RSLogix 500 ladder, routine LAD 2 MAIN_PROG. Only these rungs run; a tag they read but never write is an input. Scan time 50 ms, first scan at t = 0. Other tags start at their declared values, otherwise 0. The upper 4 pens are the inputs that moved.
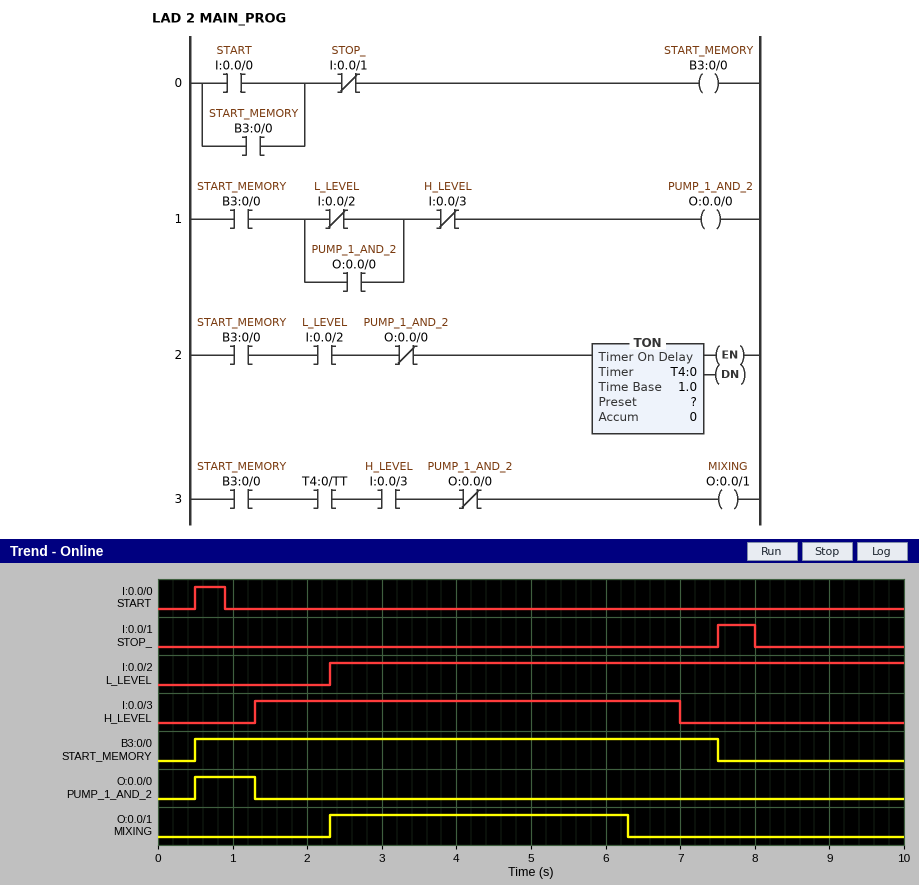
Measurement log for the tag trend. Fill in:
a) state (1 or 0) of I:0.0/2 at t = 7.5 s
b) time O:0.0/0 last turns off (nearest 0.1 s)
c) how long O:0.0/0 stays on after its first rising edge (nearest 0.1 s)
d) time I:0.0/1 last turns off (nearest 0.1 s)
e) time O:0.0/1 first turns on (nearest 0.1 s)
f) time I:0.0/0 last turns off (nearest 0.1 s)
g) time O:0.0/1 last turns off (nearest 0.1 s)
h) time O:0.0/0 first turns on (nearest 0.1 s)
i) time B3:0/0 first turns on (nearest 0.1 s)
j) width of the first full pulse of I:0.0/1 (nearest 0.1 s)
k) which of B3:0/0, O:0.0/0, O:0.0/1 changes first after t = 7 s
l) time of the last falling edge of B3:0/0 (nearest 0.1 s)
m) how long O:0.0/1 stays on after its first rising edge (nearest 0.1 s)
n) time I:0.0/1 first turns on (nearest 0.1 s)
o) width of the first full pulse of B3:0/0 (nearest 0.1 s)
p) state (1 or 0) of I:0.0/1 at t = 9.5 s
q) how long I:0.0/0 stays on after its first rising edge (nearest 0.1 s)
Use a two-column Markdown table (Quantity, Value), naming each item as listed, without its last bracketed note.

| Quantity | Value |
|---|---|
| state (1 or 0) of I:0.0/2 at t = 7.5 s | 1 |
| time O:0.0/0 last turns off | 1.3 s |
| how long O:0.0/0 stays on after its first rising edge | 0.8 s |
| time I:0.0/1 last turns off | 8.0 s |
| time O:0.0/1 first turns on | 2.3 s |
| time I:0.0/0 last turns off | 0.9 s |
| time O:0.0/1 last turns off | 6.3 s |
| time O:0.0/0 first turns on | 0.5 s |
| time B3:0/0 first turns on | 0.5 s |
| width of the first full pulse of I:0.0/1 | 0.5 s |
| which of B3:0/0, O:0.0/0, O:0.0/1 changes first after t = 7 s | B3:0/0 |
| time of the last falling edge of B3:0/0 | 7.5 s |
| how long O:0.0/1 stays on after its first rising edge | 4.0 s |
| time I:0.0/1 first turns on | 7.5 s |
| width of the first full pulse of B3:0/0 | 7.0 s |
| state (1 or 0) of I:0.0/1 at t = 9.5 s | 0 |
| how long I:0.0/0 stays on after its first rising edge | 0.4 s |
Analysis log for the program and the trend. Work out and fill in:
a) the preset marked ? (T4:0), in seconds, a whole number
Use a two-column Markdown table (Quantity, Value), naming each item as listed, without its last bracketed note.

| Quantity | Value |
|---|---|
| the preset marked ? (T4:0), in seconds, a whole number | 4 s |
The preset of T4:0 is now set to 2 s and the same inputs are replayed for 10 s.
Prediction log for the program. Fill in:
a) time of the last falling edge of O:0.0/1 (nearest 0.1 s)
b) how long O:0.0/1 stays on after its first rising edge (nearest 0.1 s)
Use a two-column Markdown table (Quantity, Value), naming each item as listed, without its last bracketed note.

| Quantity | Value |
|---|---|
| time of the last falling edge of O:0.0/1 | 4.3 s |
| how long O:0.0/1 stays on after its first rising edge | 2.0 s |
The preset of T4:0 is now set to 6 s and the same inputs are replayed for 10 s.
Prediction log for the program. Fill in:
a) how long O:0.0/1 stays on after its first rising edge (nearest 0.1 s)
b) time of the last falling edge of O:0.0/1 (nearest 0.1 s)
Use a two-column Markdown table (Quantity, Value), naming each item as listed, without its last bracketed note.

| Quantity | Value |
|---|---|
| how long O:0.0/1 stays on after its first rising edge | 4.7 s |
| time of the last falling edge of O:0.0/1 | 7.0 s |
